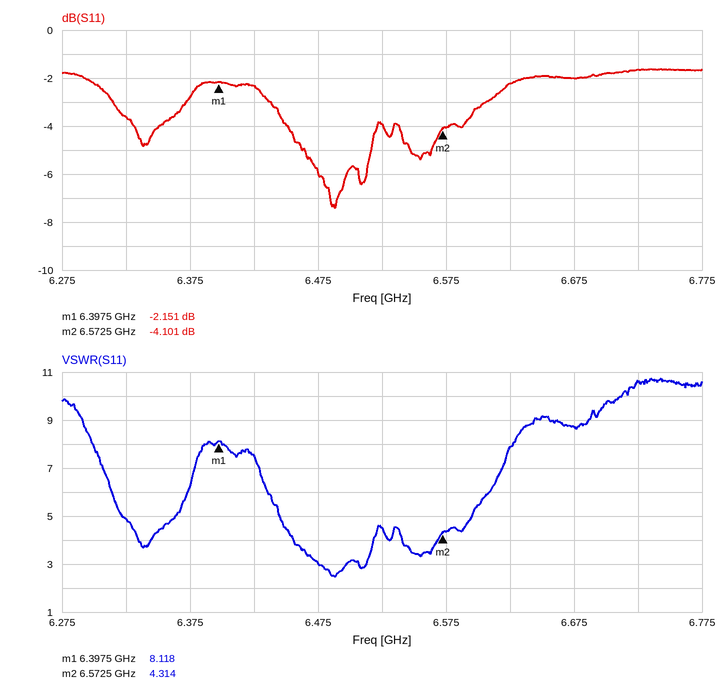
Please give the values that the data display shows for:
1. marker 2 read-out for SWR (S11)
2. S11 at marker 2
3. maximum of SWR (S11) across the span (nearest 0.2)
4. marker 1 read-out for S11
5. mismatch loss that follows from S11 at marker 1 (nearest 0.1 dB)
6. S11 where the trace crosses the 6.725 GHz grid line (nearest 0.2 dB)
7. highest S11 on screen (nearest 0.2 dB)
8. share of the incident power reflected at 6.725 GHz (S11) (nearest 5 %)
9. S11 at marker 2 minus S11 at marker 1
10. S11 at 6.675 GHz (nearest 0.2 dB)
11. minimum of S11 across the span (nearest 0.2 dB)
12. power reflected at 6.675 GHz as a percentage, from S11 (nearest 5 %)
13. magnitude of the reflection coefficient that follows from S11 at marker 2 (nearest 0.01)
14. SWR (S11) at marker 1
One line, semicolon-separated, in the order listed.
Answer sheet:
4.314; -4.101 dB; 10.8; -2.151 dB; 4.1 dB; -1.6 dB; -1.6 dB; 70 %; -1.950 dB; -2.0 dB; -7.4 dB; 65 %; 0.62; 8.118
